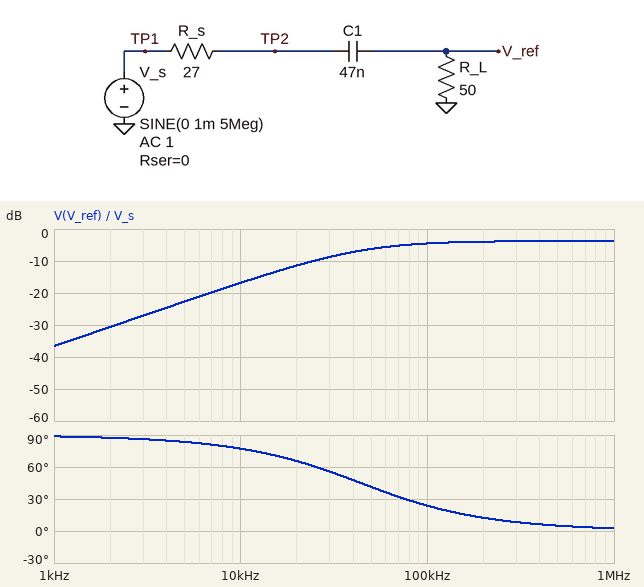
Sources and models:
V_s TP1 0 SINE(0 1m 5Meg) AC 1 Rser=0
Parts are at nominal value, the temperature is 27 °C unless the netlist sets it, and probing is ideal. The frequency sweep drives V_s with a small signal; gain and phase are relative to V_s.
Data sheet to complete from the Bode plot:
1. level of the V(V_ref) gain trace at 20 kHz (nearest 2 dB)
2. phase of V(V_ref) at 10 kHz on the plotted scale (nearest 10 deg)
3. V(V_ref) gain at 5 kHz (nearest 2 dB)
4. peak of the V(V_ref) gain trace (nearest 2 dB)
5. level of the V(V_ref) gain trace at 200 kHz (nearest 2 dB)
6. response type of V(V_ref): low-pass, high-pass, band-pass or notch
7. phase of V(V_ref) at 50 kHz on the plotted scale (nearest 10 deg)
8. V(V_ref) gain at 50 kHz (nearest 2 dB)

-12 dB
80 deg
-22 dB
-4 dB
-4 dB
high-pass
40 deg
-6 dB
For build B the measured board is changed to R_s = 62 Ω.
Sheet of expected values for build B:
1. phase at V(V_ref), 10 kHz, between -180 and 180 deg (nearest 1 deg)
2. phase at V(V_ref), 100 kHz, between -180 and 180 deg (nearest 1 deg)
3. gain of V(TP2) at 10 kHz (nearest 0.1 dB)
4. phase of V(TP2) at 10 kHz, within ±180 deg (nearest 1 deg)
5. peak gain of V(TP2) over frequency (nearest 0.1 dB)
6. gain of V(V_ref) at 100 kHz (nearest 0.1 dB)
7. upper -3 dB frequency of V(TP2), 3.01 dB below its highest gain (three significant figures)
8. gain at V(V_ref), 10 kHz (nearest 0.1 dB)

72 deg
17 deg
-0.4 dB
-10 deg
0 dB
-7.4 dB
39.0 kHz
-17.1 dB
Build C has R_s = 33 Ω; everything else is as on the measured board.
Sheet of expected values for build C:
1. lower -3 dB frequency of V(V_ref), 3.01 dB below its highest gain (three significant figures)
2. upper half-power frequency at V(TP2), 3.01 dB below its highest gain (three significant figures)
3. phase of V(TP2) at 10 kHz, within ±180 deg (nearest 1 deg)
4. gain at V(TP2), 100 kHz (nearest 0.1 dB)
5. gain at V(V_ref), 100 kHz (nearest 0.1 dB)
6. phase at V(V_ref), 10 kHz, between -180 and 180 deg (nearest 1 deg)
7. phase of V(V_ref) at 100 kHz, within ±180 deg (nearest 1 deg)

40.8 kHz
77.9 kHz
-5 deg
-3.4 dB
-5.1 dB
76 deg
22 deg
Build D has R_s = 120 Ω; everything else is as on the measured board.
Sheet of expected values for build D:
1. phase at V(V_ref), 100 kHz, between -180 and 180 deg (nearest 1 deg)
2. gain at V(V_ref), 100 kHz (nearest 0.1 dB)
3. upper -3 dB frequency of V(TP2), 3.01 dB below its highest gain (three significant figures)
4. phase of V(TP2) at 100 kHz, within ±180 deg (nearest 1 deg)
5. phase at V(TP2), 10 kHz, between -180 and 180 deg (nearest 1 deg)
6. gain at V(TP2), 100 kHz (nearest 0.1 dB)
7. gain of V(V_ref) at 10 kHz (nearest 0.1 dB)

11 deg
-10.8 dB
21.9 kHz
-23 deg
-18 deg
-9.2 dB
-17.6 dB
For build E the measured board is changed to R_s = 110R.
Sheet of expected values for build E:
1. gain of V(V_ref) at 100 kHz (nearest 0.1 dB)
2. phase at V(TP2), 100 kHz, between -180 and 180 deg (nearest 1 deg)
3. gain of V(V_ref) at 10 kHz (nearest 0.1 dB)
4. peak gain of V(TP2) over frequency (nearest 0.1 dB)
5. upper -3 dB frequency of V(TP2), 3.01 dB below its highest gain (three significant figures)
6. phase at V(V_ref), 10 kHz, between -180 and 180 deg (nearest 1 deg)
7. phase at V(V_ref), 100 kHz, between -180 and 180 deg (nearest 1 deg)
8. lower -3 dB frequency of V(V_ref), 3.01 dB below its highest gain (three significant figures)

-10.3 dB
-22 deg
-17.5 dB
0 dB
23.6 kHz
65 deg
12 deg
21.2 kHz
